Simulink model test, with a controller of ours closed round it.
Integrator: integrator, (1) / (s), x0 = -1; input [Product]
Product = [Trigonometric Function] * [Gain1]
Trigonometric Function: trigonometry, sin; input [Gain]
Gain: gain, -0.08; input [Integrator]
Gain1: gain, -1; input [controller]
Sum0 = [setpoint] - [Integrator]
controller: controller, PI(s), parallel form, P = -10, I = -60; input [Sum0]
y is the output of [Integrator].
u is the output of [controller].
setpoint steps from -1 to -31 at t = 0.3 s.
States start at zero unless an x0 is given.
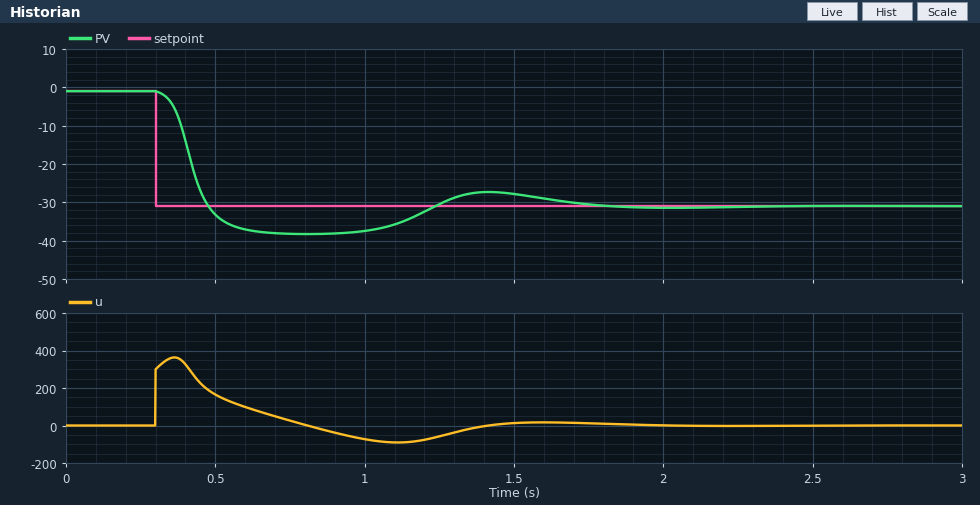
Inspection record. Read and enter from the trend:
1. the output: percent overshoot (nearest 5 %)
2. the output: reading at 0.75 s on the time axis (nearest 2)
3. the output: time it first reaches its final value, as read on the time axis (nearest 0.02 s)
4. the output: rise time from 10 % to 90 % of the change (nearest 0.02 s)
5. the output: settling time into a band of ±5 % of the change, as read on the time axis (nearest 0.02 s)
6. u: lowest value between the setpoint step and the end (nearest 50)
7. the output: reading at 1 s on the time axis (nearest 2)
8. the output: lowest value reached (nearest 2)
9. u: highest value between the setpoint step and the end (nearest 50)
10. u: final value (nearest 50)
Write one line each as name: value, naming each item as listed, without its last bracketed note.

the output: percent overshoot: 25 %
the output: reading at 0.75 s on the time axis: -38
the output: time it first reaches its final value, as read on the time axis: 0.48 s
the output: rise time from 10 % to 90 % of the change: 0.10 s
the output: settling time into a band of ±5 % of the change, as read on the time axis: 1.64 s
u: lowest value between the setpoint step and the end: -100
the output: reading at 1 s on the time axis: -38
the output: lowest value reached: -38
u: highest value between the setpoint step and the end: 350
u: final value: 0
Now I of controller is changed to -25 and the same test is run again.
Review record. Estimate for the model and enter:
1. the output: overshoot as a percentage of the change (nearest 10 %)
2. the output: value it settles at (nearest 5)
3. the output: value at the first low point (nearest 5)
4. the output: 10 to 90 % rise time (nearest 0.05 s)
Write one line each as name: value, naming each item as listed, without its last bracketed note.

the output: overshoot as a percentage of the change: 20 %
the output: value it settles at: -30
the output: value at the first low point: -35
the output: 10 to 90 % rise time: 0.15 s
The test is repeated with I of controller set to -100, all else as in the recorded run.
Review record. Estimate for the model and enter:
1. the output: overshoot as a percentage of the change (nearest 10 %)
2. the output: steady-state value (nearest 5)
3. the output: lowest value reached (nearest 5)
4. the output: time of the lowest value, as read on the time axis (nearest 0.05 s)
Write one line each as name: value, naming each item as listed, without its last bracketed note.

the output: overshoot as a percentage of the change: 30 %
the output: steady-state value: -30
the output: lowest value reached: -40
the output: time of the lowest value, as read on the time axis: 0.75 s
